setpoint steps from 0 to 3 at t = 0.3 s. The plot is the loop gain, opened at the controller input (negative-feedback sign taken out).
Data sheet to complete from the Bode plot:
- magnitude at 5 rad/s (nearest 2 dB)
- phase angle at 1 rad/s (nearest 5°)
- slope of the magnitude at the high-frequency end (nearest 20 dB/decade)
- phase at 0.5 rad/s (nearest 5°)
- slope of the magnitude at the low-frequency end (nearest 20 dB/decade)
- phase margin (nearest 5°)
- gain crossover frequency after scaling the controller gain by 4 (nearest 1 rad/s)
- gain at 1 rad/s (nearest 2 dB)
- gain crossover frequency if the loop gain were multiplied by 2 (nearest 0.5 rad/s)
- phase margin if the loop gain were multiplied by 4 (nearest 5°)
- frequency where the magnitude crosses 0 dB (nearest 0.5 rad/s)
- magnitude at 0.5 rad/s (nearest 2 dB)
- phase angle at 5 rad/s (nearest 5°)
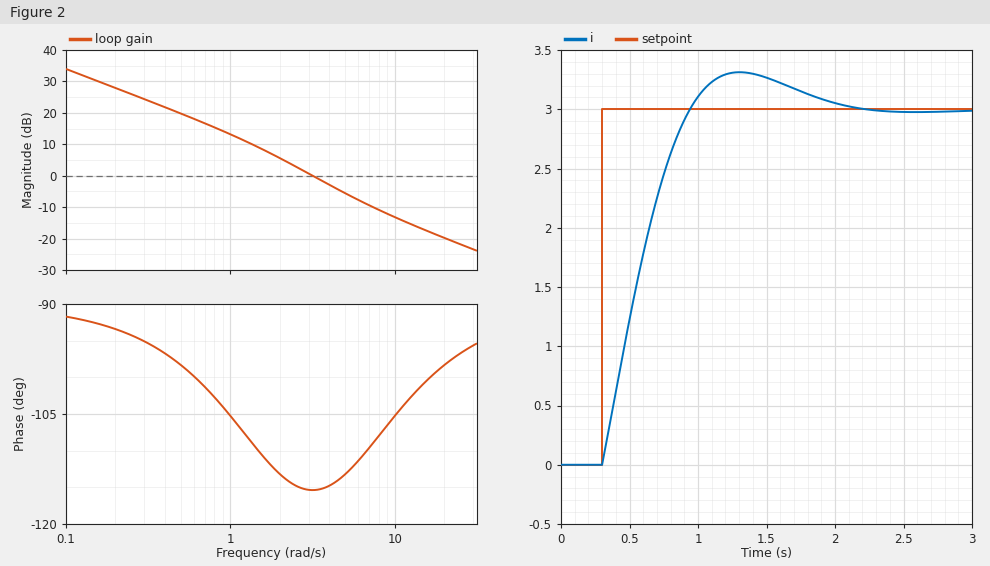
-6 dB
-105°
-20 dB/decade
-100°
-20 dB/decade
65°
9 rad/s
14 dB
5.0 rad/s
75°
3.0 rad/s
20 dB
-115°
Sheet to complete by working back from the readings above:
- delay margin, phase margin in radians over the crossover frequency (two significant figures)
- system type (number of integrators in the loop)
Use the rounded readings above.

0.38 s
1
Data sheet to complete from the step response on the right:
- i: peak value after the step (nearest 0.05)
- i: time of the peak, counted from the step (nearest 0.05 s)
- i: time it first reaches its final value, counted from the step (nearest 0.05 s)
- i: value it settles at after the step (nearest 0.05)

3.30
1.00 s
0.65 s
3.00
